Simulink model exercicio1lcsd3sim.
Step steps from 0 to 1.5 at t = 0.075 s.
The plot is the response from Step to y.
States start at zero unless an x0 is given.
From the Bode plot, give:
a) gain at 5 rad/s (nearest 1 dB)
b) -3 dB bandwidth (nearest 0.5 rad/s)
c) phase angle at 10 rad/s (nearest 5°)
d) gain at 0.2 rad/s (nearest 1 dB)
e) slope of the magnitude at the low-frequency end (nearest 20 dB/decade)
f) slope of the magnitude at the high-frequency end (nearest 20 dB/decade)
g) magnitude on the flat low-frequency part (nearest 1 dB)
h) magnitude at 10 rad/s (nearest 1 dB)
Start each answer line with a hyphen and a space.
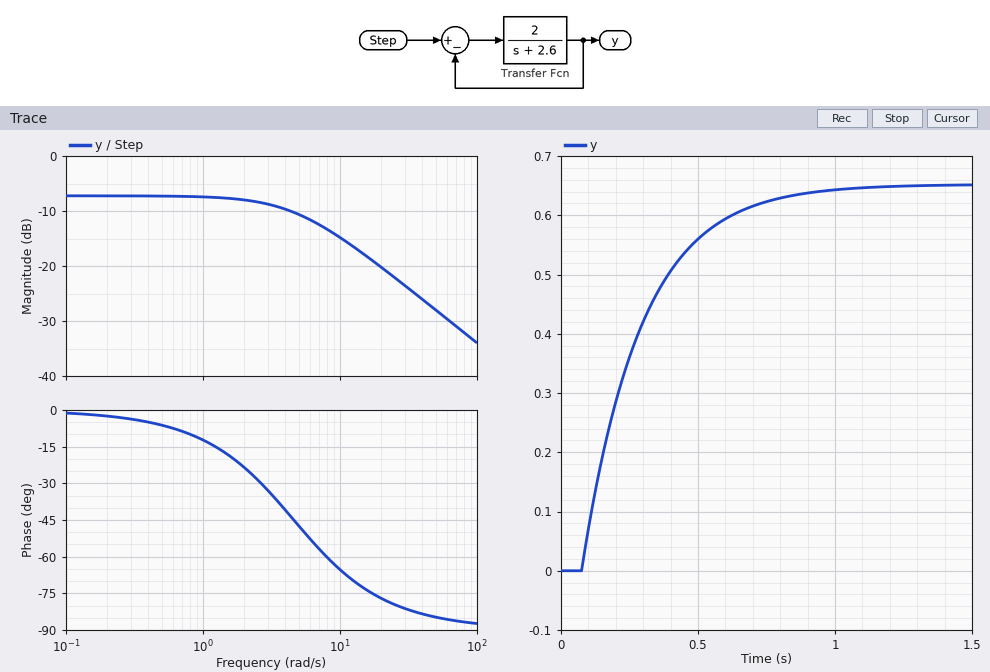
- -11 dB
- 4.5 rad/s
- -65°
- -7 dB
- 0 dB/decade
- -20 dB/decade
- -7 dB
- -15 dB
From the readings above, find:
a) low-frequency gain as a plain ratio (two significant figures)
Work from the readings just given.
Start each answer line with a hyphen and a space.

- 0.45
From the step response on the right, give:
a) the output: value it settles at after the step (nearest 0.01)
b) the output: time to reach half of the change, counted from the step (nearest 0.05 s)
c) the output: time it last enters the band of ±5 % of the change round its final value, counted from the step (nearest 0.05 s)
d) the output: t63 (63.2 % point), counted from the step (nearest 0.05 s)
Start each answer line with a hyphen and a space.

- 0.65
- 0.15 s
- 0.65 s
- 0.20 s
